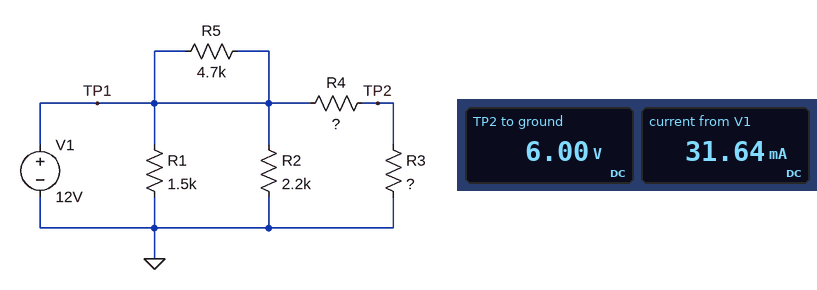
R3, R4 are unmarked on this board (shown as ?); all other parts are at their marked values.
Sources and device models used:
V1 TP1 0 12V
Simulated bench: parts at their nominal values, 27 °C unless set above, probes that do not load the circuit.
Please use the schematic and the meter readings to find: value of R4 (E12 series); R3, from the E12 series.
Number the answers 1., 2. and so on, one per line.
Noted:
1. 330 Ω
2. 330 Ω
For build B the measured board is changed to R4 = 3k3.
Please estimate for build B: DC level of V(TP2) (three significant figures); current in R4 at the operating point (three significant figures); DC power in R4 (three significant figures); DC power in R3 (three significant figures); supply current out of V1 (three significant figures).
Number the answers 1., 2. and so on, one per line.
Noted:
1. 1.09 V
2. 3.31 mA
3. 36.1 mW
4. 3.61 mW
5. 16.8 mA
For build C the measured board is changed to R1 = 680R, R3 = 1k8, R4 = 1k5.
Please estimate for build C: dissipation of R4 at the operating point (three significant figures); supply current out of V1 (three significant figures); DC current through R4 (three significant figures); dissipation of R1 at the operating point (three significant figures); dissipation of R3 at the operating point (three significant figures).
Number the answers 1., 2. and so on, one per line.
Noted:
1. 19.8 mW
2. 26.7 mA
3. 3.64 mA
4. 212 mW
5. 23.8 mW
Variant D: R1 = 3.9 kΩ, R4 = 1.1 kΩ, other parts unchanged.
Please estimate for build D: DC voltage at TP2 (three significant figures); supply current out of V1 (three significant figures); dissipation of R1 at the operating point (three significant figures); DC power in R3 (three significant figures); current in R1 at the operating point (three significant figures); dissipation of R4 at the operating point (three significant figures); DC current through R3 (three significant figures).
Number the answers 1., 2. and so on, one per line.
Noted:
1. 2.77 V
2. 16.9 mA
3. 36.9 mW
4. 23.2 mW
5. 3.08 mA
6. 77.5 mW
7. 8.39 mA
